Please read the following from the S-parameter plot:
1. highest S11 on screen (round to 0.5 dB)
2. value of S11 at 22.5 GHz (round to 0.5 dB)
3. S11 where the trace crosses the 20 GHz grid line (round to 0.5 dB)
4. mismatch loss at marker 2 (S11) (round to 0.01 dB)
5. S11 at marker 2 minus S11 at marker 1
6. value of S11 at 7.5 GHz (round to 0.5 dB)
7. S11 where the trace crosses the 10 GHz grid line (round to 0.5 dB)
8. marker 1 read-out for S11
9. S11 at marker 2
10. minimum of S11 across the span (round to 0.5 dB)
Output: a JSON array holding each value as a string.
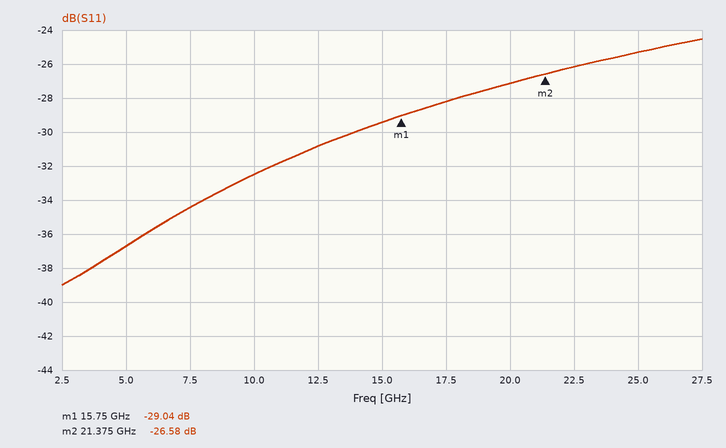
["-24.5 dB", "-26.0 dB", "-27.0 dB", "0.01 dB", "2.46 dB", "-34.5 dB", "-32.5 dB", "-29.04 dB", "-26.58 dB", "-39.0 dB"]
